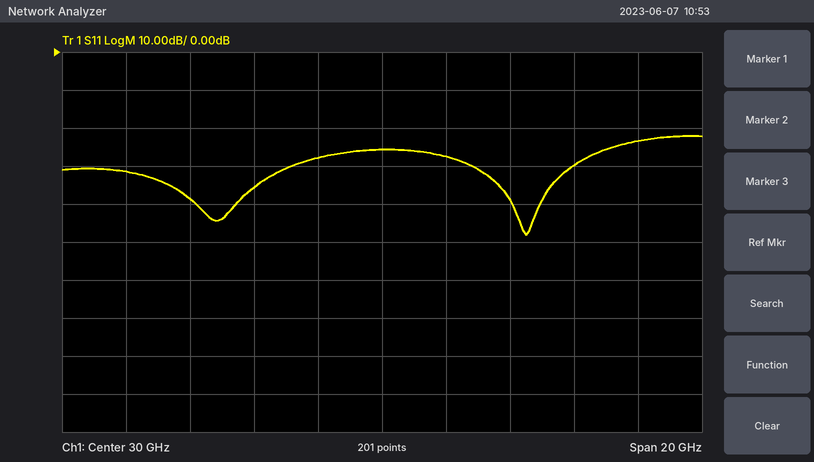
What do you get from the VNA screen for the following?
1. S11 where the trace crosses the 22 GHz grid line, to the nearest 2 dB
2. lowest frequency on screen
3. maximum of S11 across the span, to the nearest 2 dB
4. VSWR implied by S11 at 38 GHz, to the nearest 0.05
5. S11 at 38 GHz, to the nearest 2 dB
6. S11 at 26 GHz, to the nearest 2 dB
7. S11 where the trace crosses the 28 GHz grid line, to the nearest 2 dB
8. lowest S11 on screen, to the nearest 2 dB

-32 dB
20 GHz
-22 dB
1.15
-24 dB
-36 dB
-28 dB
-48 dB
